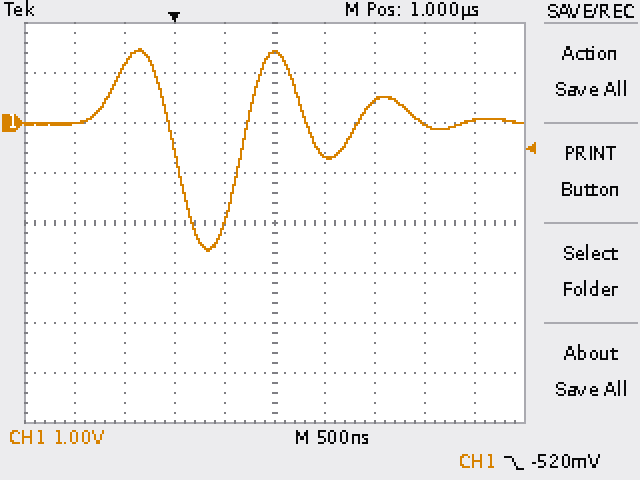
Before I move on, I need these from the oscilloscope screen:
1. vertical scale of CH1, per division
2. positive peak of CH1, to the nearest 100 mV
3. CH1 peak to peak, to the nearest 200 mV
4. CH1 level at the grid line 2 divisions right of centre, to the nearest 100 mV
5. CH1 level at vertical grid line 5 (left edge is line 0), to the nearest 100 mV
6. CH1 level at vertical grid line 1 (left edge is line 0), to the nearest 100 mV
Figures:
1 V
1.5 V
4.0 V
400 mV
1.4 V
0.0 V
